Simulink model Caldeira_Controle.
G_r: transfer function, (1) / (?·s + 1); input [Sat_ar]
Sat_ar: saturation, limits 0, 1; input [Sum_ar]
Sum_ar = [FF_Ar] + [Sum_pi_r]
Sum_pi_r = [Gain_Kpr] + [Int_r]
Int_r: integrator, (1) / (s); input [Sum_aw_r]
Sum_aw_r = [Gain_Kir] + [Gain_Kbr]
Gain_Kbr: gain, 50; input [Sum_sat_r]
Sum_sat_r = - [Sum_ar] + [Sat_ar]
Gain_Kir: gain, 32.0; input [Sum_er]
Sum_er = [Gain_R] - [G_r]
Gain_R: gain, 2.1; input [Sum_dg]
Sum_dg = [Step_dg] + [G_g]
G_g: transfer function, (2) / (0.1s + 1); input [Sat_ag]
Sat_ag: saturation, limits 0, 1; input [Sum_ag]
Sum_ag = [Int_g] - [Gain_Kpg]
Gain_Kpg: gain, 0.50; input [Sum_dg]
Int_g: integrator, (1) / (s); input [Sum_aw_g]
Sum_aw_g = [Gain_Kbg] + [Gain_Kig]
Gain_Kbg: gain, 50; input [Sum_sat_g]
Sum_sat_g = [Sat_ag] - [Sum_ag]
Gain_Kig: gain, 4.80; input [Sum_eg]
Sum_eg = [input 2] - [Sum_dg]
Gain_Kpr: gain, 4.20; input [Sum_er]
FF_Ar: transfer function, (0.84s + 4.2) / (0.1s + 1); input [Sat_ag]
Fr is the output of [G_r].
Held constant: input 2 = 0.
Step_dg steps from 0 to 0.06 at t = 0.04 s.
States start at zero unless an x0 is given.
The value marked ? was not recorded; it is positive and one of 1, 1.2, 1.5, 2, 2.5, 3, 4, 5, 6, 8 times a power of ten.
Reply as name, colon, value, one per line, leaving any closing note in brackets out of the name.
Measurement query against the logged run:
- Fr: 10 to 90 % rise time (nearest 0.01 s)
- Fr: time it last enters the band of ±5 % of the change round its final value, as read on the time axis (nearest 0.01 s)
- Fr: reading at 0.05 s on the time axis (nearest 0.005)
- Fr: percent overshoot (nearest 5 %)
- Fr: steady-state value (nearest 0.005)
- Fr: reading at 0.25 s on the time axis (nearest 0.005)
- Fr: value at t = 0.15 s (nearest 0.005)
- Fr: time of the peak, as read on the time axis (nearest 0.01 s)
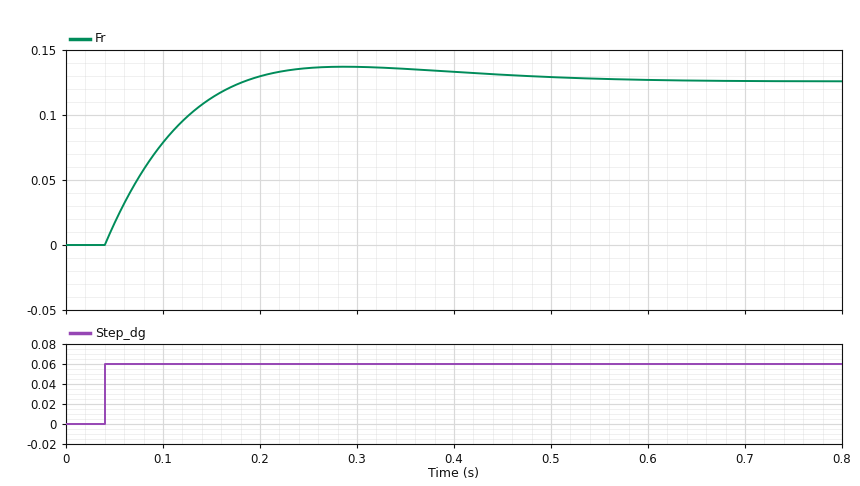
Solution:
Fr: 10 to 90 % rise time: 0.10 s
Fr: time it last enters the band of ±5 % of the change round its final value, as read on the time axis: 0.42 s
Fr: reading at 0.05 s on the time axis: 0.015
Fr: percent overshoot: 10 %
Fr: steady-state value: 0.125
Fr: reading at 0.25 s on the time axis: 0.135
Fr: value at t = 0.15 s: 0.115
Fr: time of the peak, as read on the time axis: 0.29 s
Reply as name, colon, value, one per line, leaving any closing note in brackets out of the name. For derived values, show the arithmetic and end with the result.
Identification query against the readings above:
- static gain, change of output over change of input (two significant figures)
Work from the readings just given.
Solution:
static gain, change of output over change of input: (0.125 - 0) / (0.06 - 0) = 2.1
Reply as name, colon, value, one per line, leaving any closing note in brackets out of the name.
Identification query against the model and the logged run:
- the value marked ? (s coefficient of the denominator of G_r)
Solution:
the value marked ?: 0.3
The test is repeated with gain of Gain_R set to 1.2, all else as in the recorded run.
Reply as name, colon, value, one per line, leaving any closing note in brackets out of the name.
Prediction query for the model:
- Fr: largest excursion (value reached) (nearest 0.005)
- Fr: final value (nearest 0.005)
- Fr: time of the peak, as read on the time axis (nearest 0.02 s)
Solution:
Fr: largest excursion (value reached): 0.080
Fr: final value: 0.070
Fr: time of the peak, as read on the time axis: 0.28 s
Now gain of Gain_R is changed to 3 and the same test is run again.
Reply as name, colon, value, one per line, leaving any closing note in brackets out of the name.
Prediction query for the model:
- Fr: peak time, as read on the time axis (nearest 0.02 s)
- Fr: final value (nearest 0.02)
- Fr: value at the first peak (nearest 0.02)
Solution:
Fr: peak time, as read on the time axis: 0.28 s
Fr: final value: 0.18
Fr: value at the first peak: 0.20
